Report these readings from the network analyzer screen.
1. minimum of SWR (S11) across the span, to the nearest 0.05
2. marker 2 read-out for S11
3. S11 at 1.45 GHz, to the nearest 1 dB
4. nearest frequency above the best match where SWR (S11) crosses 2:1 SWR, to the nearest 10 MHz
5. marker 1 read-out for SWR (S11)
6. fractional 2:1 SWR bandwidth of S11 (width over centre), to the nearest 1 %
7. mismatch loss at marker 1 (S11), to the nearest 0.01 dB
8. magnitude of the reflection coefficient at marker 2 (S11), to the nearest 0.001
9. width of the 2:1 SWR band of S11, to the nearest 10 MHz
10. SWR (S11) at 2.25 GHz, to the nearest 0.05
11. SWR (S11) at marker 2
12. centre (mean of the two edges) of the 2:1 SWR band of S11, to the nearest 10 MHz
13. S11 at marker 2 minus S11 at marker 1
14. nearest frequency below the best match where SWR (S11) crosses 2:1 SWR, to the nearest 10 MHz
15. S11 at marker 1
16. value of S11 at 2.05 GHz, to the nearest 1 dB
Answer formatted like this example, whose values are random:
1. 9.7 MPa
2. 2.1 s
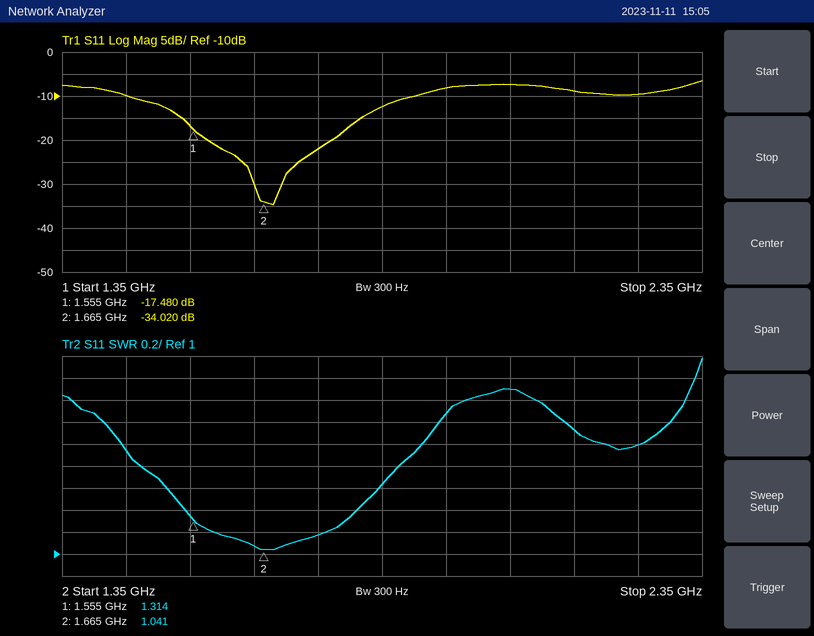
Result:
1. 1.05
2. -34.020 dB
3. -10 dB
4. 1.91 GHz
5. 1.314
6. 28 %
7. 0.08 dB
8. 0.020
9. 470 MHz
10. 2.00
11. 1.041
12. 1.68 GHz
13. -16.540 dB
14. 1.44 GHz
15. -17.480 dB
16. -7 dB
